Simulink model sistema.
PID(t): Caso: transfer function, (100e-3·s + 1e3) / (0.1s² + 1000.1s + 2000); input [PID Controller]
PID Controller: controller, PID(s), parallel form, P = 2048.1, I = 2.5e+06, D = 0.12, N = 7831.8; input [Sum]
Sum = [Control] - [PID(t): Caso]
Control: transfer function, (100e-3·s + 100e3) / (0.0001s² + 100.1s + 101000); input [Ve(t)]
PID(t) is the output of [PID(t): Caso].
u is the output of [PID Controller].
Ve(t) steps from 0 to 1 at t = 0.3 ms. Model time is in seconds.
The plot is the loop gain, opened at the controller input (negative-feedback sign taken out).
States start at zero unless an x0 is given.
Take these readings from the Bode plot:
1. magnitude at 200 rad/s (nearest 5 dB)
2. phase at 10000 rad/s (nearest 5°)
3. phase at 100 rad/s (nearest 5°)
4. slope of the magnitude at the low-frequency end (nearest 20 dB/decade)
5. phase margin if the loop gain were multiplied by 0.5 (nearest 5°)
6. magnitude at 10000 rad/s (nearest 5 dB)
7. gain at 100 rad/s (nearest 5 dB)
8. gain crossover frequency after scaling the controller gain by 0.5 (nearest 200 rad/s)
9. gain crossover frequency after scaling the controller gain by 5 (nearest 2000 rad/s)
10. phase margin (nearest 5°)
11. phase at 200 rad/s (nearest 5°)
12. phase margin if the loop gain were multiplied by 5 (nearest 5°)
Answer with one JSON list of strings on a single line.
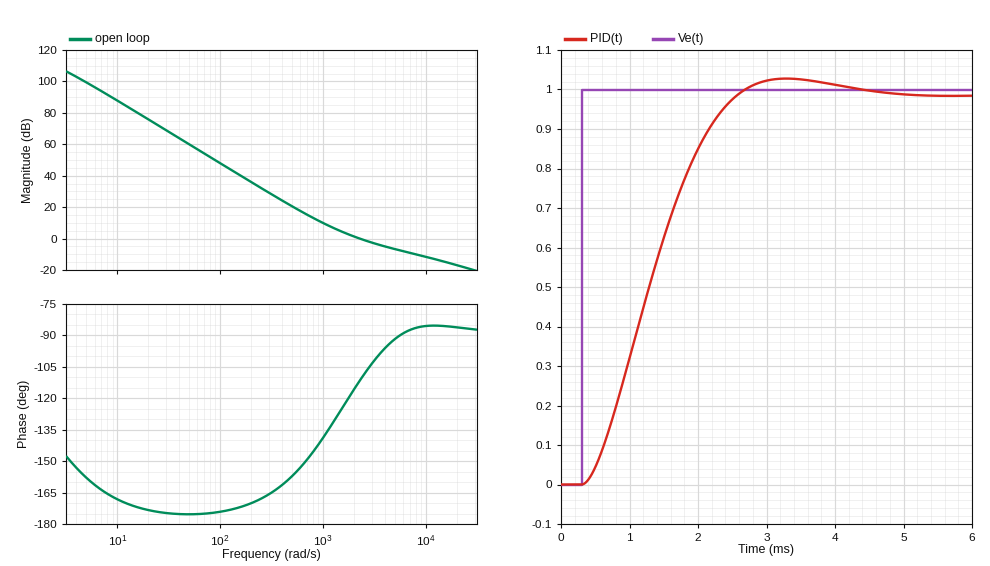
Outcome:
["35 dB", "-85°", "-175°", "-40 dB/decade", "50°", "-10 dB", "50 dB", "1400 rad/s", "14000 rad/s", "70°", "-170°", "95°"]
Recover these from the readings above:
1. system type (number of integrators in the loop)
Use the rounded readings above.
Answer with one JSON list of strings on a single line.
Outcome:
["2"]
